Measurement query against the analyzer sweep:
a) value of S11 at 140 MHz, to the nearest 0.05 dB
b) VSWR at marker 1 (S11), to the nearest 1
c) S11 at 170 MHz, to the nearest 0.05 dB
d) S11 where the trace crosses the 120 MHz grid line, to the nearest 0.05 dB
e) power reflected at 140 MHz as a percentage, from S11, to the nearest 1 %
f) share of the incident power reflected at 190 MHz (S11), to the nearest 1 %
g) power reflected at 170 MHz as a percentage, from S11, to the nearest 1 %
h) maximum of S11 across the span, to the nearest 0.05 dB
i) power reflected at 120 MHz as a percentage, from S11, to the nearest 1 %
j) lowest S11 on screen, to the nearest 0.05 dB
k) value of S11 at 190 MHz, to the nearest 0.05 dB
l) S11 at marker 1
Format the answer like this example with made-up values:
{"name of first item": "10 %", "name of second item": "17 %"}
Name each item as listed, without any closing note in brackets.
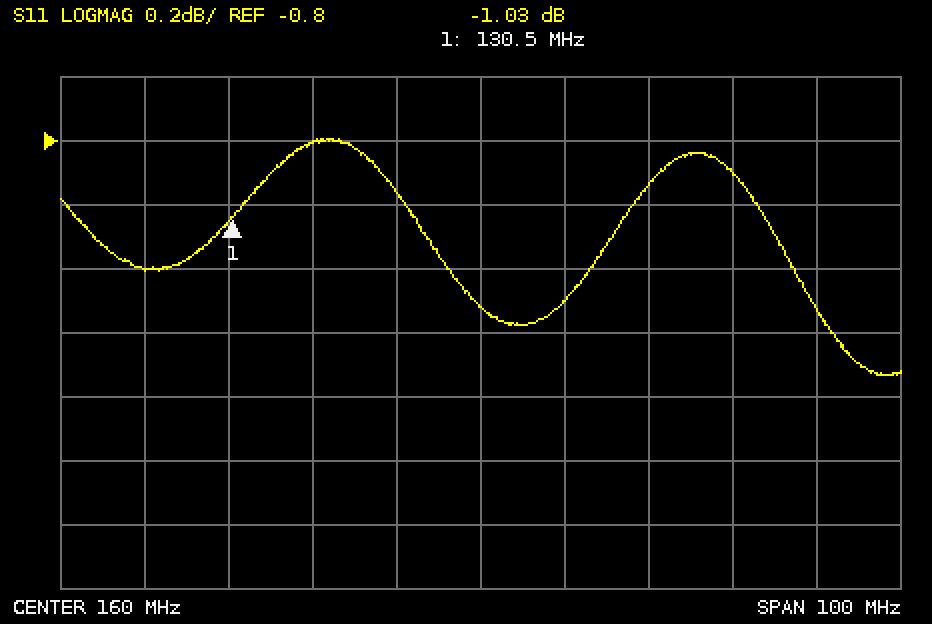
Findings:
{"value of S11 at 140 MHz, to the nearest 0.05 dB": "-0.80 dB", "VSWR at marker 1 (S11), to the nearest 1": "17", "S11 at 170 MHz, to the nearest 0.05 dB": "-1.30 dB", "S11 where the trace crosses the 120 MHz grid line, to the nearest 0.05 dB": "-1.20 dB", "power reflected at 140 MHz as a percentage, from S11, to the nearest 1 %": "83 %", "share of the incident power reflected at 190 MHz (S11), to the nearest 1 %": "81 %", "power reflected at 170 MHz as a percentage, from S11, to the nearest 1 %": "74 %", "maximum of S11 across the span, to the nearest 0.05 dB": "-0.80 dB", "power reflected at 120 MHz as a percentage, from S11, to the nearest 1 %": "76 %", "lowest S11 on screen, to the nearest 0.05 dB": "-1.55 dB", "value of S11 at 190 MHz, to the nearest 0.05 dB": "-0.90 dB", "S11 at marker 1": "-1.03 dB"}
